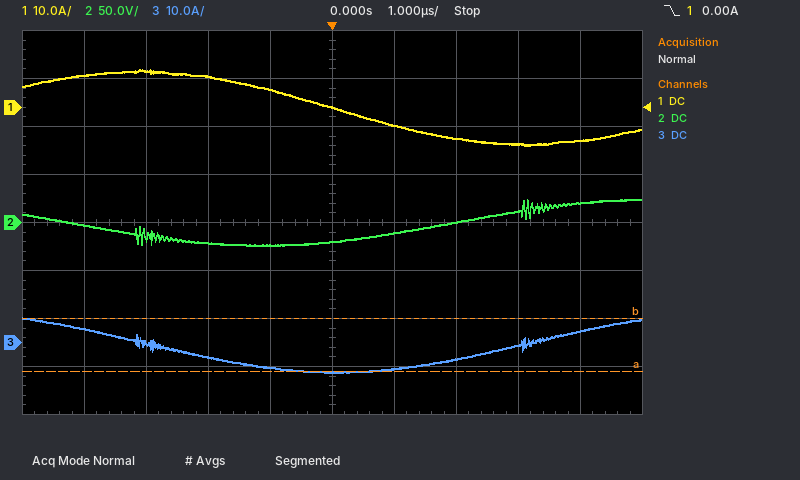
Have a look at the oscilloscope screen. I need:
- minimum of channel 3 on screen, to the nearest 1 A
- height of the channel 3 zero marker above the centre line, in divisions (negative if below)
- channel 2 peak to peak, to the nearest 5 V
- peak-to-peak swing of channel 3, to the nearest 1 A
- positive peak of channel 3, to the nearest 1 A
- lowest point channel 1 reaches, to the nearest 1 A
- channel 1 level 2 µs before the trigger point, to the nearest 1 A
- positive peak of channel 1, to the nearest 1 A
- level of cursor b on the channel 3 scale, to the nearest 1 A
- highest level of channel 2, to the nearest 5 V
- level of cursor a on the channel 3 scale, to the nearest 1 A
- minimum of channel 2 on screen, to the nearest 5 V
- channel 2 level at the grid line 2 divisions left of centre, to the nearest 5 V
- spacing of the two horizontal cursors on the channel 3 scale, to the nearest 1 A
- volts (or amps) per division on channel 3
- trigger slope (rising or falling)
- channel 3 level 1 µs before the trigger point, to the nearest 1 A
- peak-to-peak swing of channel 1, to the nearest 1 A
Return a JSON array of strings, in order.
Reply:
["-6 A", "-2.5 div", "50 V", "11 A", "5 A", "-8 A", "6 A", "8 A", "5 A", "25 V", "-6 A", "-25 V", "-20 V", "11 A", "10 A", "falling", "-5 A", "16 A"]
